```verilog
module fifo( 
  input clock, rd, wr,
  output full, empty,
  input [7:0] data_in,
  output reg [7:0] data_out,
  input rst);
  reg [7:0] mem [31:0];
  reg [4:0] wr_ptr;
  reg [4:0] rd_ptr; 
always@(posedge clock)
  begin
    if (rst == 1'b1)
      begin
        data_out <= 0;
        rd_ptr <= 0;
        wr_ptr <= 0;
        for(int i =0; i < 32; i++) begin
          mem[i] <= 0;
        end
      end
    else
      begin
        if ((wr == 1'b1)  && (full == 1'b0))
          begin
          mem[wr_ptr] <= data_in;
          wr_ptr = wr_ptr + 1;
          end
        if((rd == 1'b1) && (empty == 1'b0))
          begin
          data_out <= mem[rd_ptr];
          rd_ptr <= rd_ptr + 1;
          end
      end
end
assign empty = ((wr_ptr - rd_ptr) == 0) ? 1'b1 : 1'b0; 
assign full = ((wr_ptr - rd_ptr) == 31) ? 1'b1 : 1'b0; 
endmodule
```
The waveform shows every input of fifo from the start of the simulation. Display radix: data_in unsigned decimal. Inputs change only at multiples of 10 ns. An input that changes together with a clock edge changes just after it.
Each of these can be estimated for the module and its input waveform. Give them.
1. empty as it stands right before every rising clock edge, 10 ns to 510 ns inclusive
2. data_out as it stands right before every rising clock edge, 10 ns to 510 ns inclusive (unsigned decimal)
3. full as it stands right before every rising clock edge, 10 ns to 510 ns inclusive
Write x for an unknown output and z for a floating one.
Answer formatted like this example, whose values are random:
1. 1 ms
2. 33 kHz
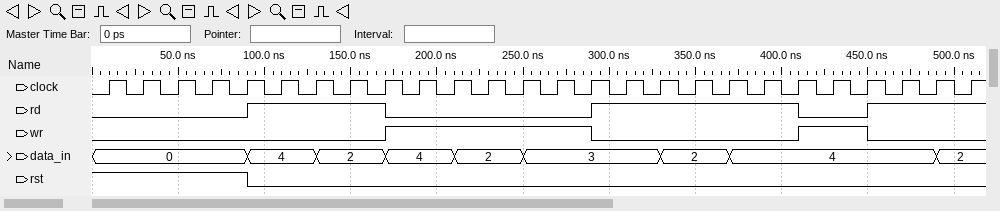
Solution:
1. x 1 1 1 1 1 1 1 1 1 0 0 0 0 0 0 0 0 0 0 0 1 0 0 0 1
2. x, 0, 0, 0, 0, 0, 0, 0, 0, 0, 0, 0, 0, 0, 0, 0, 4, 4, 2, 2, 3, 3, 3, 3, 4, 4
3. x 0 0 0 0 0 0 0 0 0 0 0 0 0 0 0 0 0 0 0 0 0 0 0 0 0
